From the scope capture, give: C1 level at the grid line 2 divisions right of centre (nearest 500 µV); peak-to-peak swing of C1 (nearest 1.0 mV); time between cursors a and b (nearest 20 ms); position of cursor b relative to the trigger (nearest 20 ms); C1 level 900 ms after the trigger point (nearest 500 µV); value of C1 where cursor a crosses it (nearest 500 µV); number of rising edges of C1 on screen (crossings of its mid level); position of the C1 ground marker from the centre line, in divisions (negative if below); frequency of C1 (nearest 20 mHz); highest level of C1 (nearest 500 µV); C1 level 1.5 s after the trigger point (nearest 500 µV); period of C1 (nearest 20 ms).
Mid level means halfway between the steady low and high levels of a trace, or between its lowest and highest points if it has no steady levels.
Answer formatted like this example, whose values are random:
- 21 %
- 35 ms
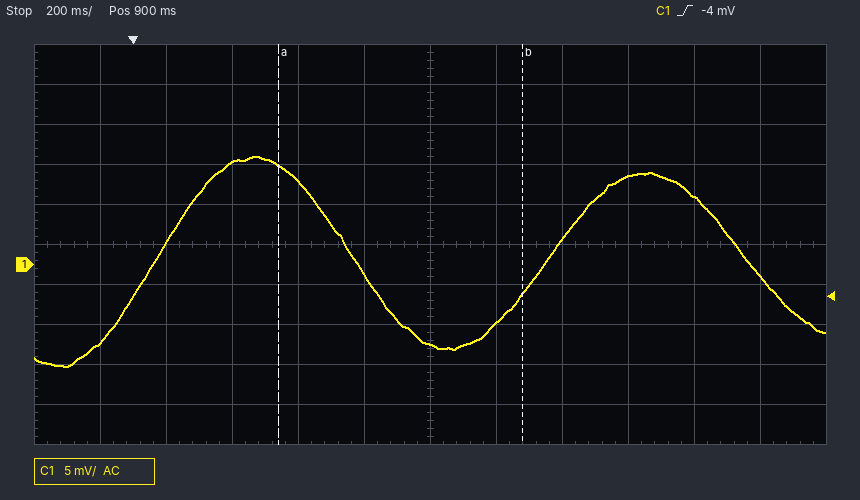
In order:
- 3.0 mV
- 26.0 mV
- 740 ms
- +1.18 s
- -10.0 mV
- 12.5 mV
- 2
- -0.5 div
- 840 mHz
- 13.5 mV
- 11.0 mV
- 1.18 s
